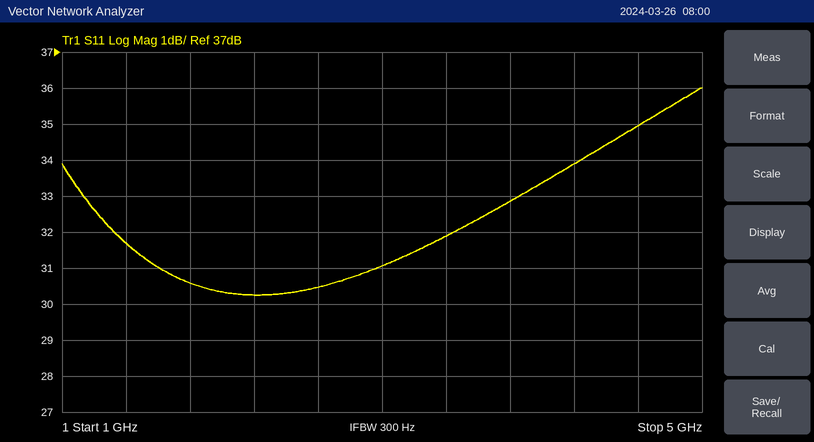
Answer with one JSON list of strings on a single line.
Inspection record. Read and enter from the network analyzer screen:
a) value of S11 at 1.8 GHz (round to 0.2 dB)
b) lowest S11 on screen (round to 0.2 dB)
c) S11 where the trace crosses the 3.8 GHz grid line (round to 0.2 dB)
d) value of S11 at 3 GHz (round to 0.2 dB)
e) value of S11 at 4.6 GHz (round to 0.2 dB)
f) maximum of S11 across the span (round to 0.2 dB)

["30.6 dB", "30.2 dB", "32.8 dB", "31.0 dB", "35.0 dB", "36.0 dB"]
